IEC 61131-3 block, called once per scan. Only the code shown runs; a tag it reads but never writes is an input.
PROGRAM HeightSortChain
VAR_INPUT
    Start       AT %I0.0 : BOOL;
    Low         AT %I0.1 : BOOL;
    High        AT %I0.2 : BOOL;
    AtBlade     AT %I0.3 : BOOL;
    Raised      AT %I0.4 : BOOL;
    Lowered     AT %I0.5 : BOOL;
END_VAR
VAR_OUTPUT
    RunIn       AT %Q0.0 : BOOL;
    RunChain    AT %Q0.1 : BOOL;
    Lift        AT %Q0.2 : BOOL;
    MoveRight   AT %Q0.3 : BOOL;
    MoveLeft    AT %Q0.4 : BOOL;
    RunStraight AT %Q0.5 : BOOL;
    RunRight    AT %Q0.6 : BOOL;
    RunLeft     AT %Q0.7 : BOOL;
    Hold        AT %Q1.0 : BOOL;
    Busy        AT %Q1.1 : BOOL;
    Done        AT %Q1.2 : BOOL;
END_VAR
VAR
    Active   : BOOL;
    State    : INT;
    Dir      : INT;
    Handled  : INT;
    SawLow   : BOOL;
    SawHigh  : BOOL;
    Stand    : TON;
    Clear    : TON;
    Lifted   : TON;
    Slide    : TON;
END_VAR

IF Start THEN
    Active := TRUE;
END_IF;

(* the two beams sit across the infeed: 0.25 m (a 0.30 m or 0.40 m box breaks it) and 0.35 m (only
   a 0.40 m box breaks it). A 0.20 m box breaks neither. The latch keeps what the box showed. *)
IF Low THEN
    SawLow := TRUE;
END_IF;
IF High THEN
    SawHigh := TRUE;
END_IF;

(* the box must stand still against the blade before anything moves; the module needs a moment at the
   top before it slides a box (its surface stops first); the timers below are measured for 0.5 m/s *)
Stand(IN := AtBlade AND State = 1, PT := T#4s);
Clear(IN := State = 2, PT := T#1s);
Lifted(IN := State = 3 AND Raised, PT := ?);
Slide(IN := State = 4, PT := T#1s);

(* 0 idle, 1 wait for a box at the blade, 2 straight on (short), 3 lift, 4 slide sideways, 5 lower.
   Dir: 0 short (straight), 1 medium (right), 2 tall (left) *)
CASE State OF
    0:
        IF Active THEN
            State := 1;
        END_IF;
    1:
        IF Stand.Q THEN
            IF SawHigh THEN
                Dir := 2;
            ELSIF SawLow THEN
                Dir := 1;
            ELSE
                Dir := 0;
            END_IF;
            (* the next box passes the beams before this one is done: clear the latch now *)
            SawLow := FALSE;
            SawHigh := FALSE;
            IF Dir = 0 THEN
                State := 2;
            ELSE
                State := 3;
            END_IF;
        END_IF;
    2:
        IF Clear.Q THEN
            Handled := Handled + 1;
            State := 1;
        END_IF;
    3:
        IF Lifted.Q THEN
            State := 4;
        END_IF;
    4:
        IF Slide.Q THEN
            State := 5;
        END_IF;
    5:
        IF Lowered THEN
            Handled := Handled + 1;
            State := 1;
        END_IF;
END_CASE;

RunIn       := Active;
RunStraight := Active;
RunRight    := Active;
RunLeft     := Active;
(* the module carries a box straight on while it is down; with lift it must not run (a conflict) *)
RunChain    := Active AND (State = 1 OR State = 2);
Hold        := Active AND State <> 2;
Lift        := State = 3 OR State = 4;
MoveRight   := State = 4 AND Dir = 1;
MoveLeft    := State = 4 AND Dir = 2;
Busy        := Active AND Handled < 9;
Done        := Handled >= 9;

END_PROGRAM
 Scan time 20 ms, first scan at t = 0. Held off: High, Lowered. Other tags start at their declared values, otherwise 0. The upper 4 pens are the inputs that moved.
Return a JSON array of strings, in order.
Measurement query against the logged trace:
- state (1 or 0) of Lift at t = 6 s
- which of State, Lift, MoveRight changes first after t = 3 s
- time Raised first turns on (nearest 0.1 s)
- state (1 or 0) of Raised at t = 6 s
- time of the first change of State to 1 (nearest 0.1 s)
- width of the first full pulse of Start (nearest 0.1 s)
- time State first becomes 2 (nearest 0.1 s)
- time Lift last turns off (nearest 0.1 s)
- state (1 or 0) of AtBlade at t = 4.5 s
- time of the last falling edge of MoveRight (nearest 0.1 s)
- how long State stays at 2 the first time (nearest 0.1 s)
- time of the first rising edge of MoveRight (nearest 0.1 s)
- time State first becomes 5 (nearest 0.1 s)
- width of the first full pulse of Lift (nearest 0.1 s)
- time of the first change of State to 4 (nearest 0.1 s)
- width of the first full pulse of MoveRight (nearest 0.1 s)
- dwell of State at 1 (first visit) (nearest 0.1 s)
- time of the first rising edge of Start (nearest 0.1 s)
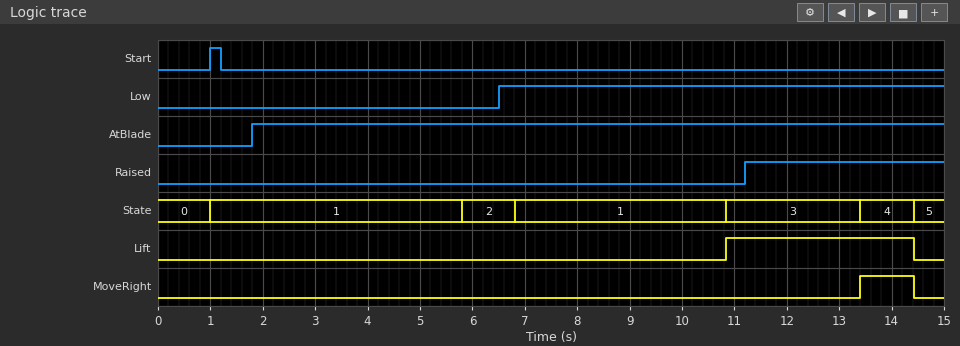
["0", "State", "11.2 s", "0", "1.0 s", "0.2 s", "5.8 s", "14.4 s", "1", "14.4 s", "1.0 s", "13.4 s", "14.4 s", "3.6 s", "13.4 s", "1.0 s", "4.8 s", "1.0 s"]
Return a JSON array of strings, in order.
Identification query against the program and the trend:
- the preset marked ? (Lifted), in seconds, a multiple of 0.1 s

["2.2 s"]
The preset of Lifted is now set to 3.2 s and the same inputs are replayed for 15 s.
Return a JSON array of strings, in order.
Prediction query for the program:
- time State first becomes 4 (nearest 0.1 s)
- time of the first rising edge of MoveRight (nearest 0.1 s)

["14.4 s", "14.4 s"]
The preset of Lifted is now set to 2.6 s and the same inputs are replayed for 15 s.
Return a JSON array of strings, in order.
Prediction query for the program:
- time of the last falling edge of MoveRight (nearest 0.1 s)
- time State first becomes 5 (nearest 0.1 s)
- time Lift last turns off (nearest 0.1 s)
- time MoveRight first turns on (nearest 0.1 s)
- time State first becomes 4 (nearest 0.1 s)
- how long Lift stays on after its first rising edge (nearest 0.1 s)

["14.8 s", "14.8 s", "14.8 s", "13.8 s", "13.8 s", "4.0 s"]
